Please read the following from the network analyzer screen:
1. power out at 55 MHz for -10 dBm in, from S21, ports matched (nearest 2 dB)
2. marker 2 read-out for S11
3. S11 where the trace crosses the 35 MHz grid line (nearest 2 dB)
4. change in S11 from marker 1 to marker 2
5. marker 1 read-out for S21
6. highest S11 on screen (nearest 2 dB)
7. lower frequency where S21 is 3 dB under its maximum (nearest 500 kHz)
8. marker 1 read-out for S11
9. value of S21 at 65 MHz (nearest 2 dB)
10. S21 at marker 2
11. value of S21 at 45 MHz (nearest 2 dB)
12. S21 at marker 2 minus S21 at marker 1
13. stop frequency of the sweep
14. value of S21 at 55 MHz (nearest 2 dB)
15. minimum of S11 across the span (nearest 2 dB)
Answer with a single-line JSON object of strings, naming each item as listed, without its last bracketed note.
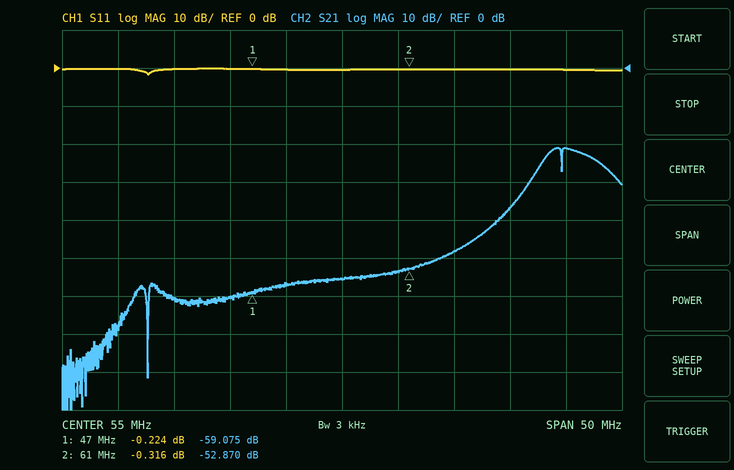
{"power out at 55 MHz for -10 dBm in, from S21, ports matched": "-66 dBm", "marker 2 read-out for S11": "-0.316 dB", "S11 where the trace crosses the 35 MHz grid line": "0 dB", "change in S11 from marker 1 to marker 2": "-0.092 dB", "marker 1 read-out for S21": "-59.075 dB", "highest S11 on screen": "0 dB", "lower frequency where S21 is 3 dB under its maximum": "73.0 MHz", "marker 1 read-out for S11": "-0.224 dB", "value of S21 at 65 MHz": "-48 dB", "S21 at marker 2": "-52.870 dB", "value of S21 at 45 MHz": "-60 dB", "S21 at marker 2 minus S21 at marker 1": "6.205 dB", "stop frequency of the sweep": "80 MHz", "value of S21 at 55 MHz": "-56 dB", "minimum of S11 across the span": "-2 dB"}
